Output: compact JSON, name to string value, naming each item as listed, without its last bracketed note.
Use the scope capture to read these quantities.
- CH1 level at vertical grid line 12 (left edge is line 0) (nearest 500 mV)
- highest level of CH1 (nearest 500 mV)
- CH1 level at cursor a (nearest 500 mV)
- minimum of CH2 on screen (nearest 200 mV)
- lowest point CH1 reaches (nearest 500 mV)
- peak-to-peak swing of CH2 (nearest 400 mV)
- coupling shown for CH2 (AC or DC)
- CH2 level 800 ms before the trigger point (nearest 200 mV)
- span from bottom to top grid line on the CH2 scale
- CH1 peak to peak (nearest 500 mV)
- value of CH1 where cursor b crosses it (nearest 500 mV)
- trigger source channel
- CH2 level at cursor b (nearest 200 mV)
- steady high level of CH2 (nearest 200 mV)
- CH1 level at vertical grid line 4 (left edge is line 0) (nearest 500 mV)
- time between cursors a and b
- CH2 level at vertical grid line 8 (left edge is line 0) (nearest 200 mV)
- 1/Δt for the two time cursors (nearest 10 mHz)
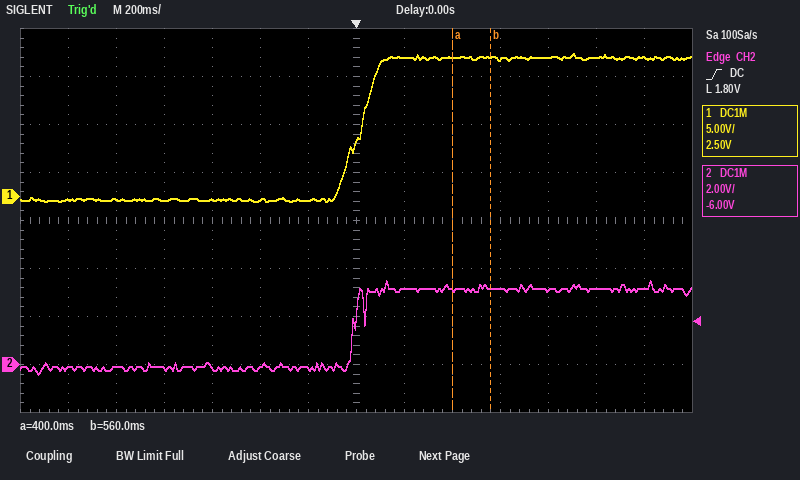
{"CH1 level at vertical grid line 12 (left edge is line 0)": "14.5 V", "highest level of CH1": "15.0 V", "CH1 level at cursor a": "14.5 V", "minimum of CH2 on screen": "-400 mV", "lowest point CH1 reaches": "-500 mV", "peak-to-peak swing of CH2": "4.0 V", "coupling shown for CH2": "DC", "CH2 level 800 ms before the trigger point": "-200 mV", "span from bottom to top grid line on the CH2 scale": "16 V", "CH1 peak to peak": "15.5 V", "value of CH1 where cursor b crosses it": "14.5 V", "trigger source channel": "CH2", "CH2 level at cursor b": "3.2 V", "steady high level of CH2": "3.2 V", "CH1 level at vertical grid line 4 (left edge is line 0)": "-500 mV", "time between cursors a and b": "160 ms", "CH2 level at vertical grid line 8 (left edge is line 0)": "3.2 V", "1/Δt for the two time cursors": "6.25 Hz"}
